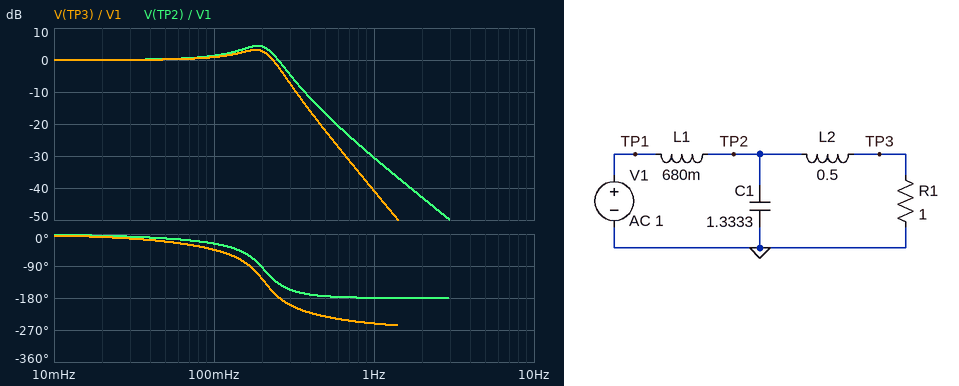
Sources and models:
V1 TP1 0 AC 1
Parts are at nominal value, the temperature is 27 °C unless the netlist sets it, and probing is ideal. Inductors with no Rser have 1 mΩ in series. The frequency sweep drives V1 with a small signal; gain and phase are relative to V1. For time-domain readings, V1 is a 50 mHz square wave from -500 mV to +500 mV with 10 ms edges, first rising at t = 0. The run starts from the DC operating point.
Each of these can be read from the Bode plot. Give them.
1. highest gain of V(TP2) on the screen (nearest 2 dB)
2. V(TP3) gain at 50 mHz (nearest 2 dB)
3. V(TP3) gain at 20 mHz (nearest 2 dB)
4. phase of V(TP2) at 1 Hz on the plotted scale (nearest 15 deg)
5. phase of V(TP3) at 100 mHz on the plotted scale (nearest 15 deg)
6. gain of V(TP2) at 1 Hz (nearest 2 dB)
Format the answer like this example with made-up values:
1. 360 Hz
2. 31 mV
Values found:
1. 4 dB
2. 0 dB
3. 0 dB
4. -180 deg
5. -45 deg
6. -30 dB
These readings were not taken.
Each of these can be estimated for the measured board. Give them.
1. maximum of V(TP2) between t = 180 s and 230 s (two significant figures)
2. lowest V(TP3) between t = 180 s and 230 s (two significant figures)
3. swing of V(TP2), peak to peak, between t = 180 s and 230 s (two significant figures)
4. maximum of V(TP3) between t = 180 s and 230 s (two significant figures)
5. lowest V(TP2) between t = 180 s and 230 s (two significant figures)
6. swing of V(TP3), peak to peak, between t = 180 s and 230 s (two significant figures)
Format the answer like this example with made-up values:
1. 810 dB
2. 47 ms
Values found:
1. 810 mV
2. -750 mV
3. 1.6 V
4. 750 mV
5. -810 mV
6. 1.5 V
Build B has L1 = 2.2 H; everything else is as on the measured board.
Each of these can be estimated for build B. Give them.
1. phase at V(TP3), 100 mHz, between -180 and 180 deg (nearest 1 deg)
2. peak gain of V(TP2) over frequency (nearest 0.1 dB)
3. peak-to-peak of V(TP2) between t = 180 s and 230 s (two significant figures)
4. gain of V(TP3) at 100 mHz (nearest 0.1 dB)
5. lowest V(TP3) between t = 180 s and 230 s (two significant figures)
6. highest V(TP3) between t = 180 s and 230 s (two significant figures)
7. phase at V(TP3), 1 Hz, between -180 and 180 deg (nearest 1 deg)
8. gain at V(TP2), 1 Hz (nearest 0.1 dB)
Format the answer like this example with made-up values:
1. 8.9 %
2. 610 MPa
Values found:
1. -97 deg
2. 0 dB
3. 1.0 V
4. -2.6 dB
5. -510 mV
6. 510 mV
7. 108 deg
8. -40.9 dB
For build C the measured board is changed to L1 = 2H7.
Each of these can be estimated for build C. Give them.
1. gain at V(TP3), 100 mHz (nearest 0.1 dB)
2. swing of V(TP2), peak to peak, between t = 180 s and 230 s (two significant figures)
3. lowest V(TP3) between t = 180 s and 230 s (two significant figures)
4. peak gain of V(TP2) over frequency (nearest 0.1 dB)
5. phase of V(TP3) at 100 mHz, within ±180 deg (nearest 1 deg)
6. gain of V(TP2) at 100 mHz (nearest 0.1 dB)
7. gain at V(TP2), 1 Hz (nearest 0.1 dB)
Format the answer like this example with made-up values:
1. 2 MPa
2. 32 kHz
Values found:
1. -4.2 dB
2. 990 mV
3. -490 mV
4. 0 dB
5. -105 deg
6. -3.8 dB
7. -42.7 dB
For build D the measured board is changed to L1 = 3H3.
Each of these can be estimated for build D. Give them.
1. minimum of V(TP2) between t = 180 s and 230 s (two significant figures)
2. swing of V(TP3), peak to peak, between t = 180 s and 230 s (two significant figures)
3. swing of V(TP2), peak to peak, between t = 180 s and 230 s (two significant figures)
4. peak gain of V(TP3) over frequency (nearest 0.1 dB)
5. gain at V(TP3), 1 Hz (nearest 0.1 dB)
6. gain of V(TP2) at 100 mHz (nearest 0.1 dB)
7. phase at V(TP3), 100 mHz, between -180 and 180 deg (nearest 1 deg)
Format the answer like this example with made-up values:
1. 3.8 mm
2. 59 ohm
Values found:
1. -480 mV
2. 950 mV
3. 960 mV
4. 0 dB
5. -54.8 dB
6. -5.5 dB
7. -112 deg
